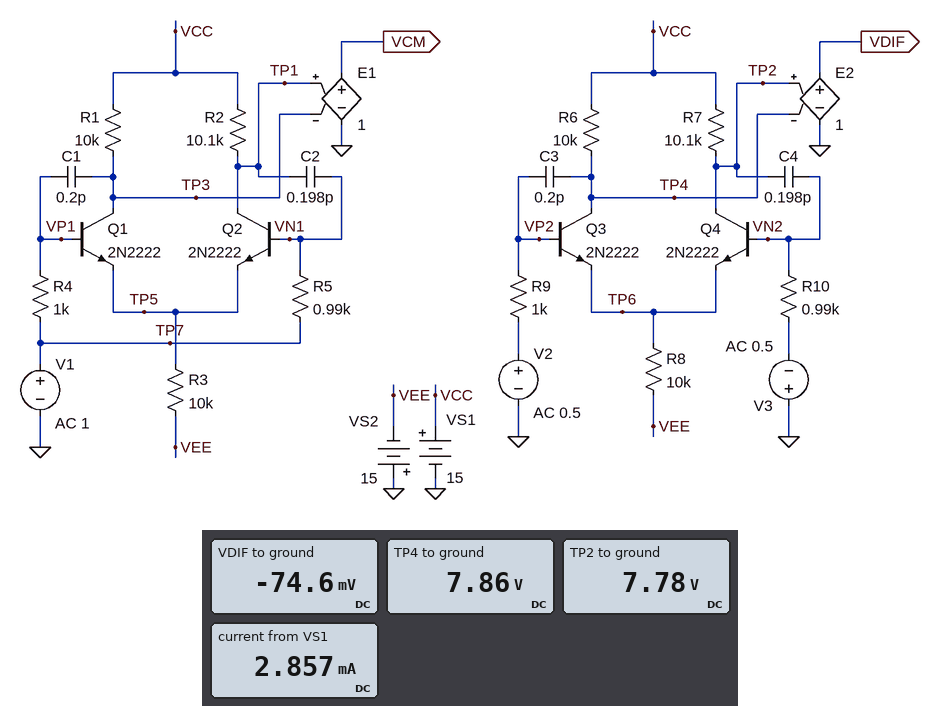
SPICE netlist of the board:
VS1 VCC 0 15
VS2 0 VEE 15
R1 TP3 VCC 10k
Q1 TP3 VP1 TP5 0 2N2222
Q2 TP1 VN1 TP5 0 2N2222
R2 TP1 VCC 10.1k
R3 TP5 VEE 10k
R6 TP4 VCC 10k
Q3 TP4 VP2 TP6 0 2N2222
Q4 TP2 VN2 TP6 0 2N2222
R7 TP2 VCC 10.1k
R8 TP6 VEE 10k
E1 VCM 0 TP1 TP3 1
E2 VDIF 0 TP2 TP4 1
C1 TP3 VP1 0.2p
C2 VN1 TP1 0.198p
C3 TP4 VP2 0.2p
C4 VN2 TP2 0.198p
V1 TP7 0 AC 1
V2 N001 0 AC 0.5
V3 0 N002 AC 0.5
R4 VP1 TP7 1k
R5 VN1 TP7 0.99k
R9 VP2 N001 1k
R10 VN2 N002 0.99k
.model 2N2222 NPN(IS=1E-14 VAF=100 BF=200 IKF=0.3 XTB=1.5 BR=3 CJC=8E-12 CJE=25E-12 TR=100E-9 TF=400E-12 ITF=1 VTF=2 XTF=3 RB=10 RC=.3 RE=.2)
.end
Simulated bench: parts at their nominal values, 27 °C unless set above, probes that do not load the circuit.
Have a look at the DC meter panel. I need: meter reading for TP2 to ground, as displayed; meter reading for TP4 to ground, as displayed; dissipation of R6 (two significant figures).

7.78 V
7.86 V
5.1 mW
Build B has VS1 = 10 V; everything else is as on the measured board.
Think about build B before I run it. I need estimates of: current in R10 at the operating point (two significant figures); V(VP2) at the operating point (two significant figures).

3.5 µA
-3.5 mV
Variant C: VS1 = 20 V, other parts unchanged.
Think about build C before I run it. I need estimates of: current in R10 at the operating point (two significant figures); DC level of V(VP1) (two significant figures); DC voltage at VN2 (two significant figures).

3.2 µA
-3.2 mV
-3.1 mV
